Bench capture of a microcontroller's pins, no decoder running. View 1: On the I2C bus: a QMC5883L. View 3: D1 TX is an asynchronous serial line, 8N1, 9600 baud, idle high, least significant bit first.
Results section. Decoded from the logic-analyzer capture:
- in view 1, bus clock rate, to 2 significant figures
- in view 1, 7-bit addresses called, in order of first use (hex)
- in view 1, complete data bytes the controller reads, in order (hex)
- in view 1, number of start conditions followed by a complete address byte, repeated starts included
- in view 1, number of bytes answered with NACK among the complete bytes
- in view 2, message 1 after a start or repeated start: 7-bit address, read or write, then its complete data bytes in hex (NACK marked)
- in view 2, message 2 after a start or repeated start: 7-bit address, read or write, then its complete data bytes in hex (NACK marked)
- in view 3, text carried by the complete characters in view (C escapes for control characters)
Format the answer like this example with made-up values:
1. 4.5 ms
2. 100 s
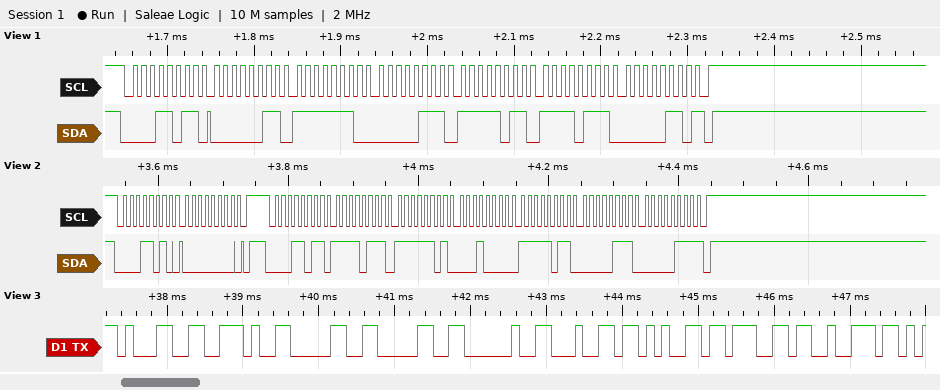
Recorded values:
1. 100 kHz
2. 0x0D
3. 03 FE 07 FB F7 06
4. 1
5. 1
6. 0x0D write: 00
7. 0x0D read: F7 FD 10 FB 07 07 NACK
8. "1.00 degr"
